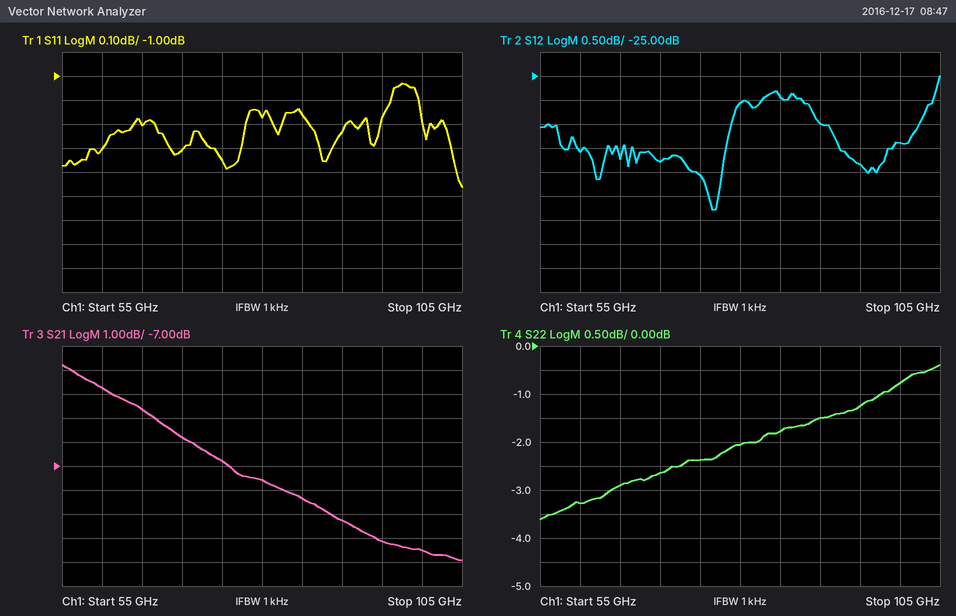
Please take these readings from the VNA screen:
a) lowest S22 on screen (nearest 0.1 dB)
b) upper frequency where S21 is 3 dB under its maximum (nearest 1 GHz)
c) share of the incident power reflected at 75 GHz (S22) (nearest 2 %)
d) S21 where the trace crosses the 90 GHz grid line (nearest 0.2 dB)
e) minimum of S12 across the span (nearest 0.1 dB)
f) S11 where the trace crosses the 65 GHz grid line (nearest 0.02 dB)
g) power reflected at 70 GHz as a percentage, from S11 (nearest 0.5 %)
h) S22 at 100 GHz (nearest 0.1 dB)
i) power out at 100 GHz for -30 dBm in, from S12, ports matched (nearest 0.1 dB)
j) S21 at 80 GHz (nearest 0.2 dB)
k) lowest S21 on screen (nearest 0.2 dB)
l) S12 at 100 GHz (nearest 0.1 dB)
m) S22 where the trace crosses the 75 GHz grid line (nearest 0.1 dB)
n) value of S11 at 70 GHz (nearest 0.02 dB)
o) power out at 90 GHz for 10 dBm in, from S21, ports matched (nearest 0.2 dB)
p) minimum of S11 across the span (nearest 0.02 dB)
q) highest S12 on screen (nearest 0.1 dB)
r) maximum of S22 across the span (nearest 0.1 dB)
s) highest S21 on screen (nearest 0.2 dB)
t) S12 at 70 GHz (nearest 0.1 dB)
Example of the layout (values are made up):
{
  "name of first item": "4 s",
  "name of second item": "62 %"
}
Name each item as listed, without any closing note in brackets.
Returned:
{
  "lowest S22 on screen": "-3.6 dB",
  "upper frequency where S21 is 3 dB under its maximum": "70 GHz",
  "share of the incident power reflected at 75 GHz (S22)": "58 %",
  "S21 where the trace crosses the 90 GHz grid line": "-9.2 dB",
  "minimum of S12 across the span": "-27.8 dB",
  "S11 where the trace crosses the 65 GHz grid line": "-1.20 dB",
  "power reflected at 70 GHz as a percentage, from S11": "74.0 %",
  "S22 at 100 GHz": "-0.8 dB",
  "power out at 100 GHz for -30 dBm in, from S12, ports matched": "-56.4 dBm",
  "S21 at 80 GHz": "-7.6 dB",
  "lowest S21 on screen": "-11.0 dB",
  "S12 at 100 GHz": "-26.4 dB",
  "S22 where the trace crosses the 75 GHz grid line": "-2.4 dB",
  "value of S11 at 70 GHz": "-1.30 dB",
  "power out at 90 GHz for 10 dBm in, from S21, ports matched": "0.8 dBm",
  "minimum of S11 across the span": "-1.46 dB",
  "highest S12 on screen": "-25.0 dB",
  "maximum of S22 across the span": "-0.4 dB",
  "highest S21 on screen": "-2.8 dB",
  "S12 at 70 GHz": "-26.8 dB"
}
